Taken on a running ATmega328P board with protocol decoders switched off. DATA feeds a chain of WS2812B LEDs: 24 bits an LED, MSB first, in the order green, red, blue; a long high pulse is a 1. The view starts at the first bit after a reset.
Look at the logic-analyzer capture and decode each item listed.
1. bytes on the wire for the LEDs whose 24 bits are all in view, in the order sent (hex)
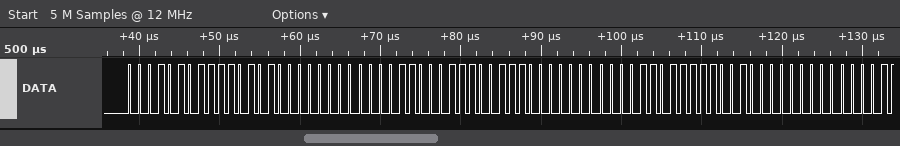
15 EA 00 18 E7 00 1B E4 00
